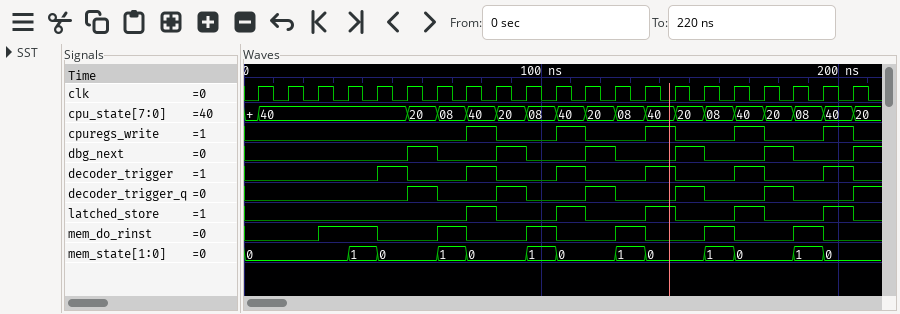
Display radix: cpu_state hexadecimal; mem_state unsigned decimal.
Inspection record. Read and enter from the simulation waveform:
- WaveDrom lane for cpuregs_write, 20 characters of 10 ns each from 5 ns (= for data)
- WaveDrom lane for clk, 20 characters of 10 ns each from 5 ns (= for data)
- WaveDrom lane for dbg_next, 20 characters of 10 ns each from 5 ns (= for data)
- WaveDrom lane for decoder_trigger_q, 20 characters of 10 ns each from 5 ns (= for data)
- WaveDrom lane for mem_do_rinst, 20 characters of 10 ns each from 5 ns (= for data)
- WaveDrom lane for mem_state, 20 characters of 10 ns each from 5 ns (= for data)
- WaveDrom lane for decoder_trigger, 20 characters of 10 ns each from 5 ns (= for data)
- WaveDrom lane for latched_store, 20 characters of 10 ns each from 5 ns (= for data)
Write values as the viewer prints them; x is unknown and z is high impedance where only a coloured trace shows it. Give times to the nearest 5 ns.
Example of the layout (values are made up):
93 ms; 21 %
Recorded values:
{name: 'cpuregs_write', wave: '0......10.10.10.10.1'}; {name: 'clk', wave: 'p...................'}; {name: 'dbg_next', wave: '0....10.10.10.10.10.'}; {name: 'decoder_trigger_q', wave: '0....10.10.10.10.10.'}; {name: 'mem_do_rinst', wave: '0.1.0.10.10.10.10.10'}; {name: 'mem_state', wave: '=..==.==.==.==.==.==', data: '0 1 0 1 0 1 0 1 0 1 0 1 0'}; {name: 'decoder_trigger', wave: '0...10.10.10.10.10.1'}; {name: 'latched_store', wave: '0......10.10.10.10.1'}
